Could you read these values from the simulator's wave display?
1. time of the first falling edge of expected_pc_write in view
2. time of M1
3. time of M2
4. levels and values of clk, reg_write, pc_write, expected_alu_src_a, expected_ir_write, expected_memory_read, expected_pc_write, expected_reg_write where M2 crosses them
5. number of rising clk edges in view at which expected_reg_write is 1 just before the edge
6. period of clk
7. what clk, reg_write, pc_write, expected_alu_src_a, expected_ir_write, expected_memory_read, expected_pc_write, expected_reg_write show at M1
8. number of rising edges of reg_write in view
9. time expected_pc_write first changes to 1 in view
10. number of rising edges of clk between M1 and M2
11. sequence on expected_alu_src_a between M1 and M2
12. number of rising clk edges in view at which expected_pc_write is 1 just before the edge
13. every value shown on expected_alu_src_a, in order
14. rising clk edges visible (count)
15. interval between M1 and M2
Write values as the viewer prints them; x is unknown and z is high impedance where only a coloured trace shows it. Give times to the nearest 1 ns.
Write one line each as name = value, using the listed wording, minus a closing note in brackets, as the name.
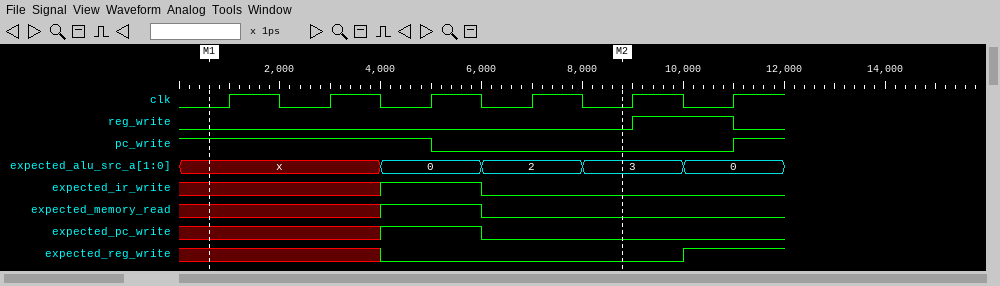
time of the first falling edge of expected_pc_write in view = 6 ns
time of M1 = 1 ns
time of M2 = 9 ns
levels and values of clk, reg_write, pc_write, expected_alu_src_a, expected_ir_write, expected_memory_read, expected_pc_write, expected_reg_write where M2 crosses them = clk=0, reg_write=0, pc_write=0, expected_alu_src_a=3, expected_ir_write=0, expected_memory_read=0, expected_pc_write=0, expected_reg_write=0
number of rising clk edges in view at which expected_reg_write is 1 just before the edge = 1
period of clk = 2 ns
what clk, reg_write, pc_write, expected_alu_src_a, expected_ir_write, expected_memory_read, expected_pc_write, expected_reg_write show at M1 = clk=0, reg_write=0, pc_write=1, expected_alu_src_a=x, expected_ir_write=x, expected_memory_read=x, expected_pc_write=x, expected_reg_write=x
number of rising edges of reg_write in view = 1
time expected_pc_write first changes to 1 in view = 4 ns
number of rising edges of clk between M1 and M2 = 4
sequence on expected_alu_src_a between M1 and M2 = x, 0, 2, 3
number of rising clk edges in view at which expected_pc_write is 1 just before the edge = 1
every value shown on expected_alu_src_a, in order = x, 0, 2, 3, 0
rising clk edges visible = 6
interval between M1 and M2 = 8 ns
